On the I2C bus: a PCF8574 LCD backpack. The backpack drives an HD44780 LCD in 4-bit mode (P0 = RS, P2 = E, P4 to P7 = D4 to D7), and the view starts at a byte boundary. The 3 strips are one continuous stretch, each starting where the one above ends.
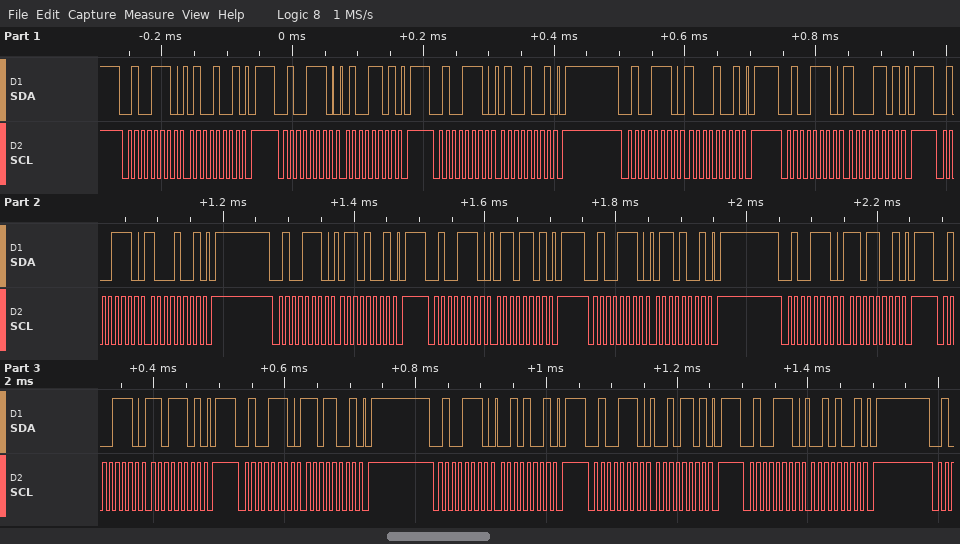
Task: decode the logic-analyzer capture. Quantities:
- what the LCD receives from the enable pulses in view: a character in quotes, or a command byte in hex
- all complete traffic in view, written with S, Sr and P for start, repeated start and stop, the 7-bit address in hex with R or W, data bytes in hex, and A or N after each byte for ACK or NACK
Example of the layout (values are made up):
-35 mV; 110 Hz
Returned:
'H' 'm'; S 27W A 49 A P S 27W A 4D A P S 27W A 49 A P S 27W A 89 A P S 27W A 8D A P S 27W A 89 A P S 27W A 69 A P S 27W A 6D A P S 27W A 69 A P S 27W A D9 A P S 27W A DD A P S 27W A D9 A P S 27W A 29 A P S 27W A 2D A P S 27W A 29 A P
